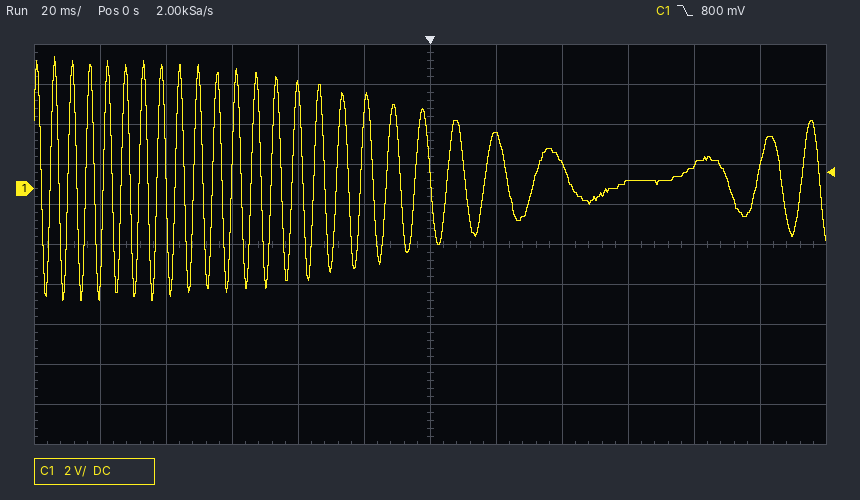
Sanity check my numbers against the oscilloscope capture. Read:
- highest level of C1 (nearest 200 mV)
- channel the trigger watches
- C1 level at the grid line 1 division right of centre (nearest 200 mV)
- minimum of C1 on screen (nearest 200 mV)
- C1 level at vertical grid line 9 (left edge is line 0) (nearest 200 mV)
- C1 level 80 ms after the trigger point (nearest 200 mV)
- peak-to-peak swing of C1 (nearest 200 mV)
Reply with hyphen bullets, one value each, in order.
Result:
- 6.6 V
- C1
- 2.6 V
- -5.6 V
- 400 mV
- 1.2 V
- 12.2 V
